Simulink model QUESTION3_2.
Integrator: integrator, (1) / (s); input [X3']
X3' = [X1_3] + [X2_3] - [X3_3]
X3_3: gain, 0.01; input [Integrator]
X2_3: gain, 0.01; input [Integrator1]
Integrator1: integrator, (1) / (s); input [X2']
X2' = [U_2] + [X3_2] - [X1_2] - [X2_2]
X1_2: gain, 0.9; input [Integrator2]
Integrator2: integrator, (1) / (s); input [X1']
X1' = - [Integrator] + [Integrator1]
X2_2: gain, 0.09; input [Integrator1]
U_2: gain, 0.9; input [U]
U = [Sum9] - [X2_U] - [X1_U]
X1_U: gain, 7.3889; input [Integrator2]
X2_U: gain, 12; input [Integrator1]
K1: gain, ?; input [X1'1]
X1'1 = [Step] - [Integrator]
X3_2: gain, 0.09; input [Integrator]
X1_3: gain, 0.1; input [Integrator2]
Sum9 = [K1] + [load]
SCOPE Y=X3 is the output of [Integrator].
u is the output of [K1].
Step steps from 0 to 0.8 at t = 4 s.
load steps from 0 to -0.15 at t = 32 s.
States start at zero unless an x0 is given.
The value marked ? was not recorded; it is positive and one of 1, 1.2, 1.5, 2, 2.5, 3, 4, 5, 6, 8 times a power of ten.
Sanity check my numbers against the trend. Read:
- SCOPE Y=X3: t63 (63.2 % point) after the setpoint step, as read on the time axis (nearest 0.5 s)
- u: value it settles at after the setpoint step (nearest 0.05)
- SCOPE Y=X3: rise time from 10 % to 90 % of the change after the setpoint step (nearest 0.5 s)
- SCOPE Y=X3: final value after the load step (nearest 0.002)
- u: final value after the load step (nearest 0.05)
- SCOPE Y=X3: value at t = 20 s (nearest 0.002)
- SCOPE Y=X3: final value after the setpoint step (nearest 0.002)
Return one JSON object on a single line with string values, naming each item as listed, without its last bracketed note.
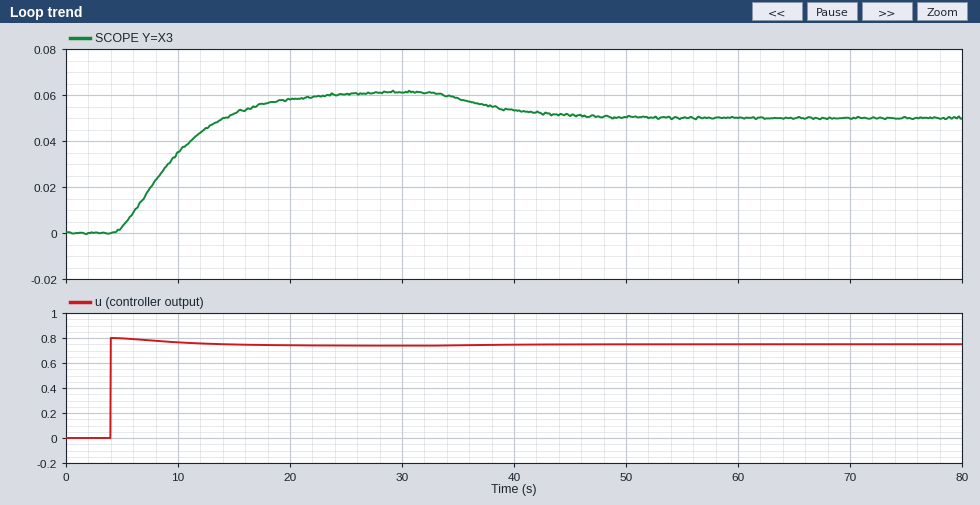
{"SCOPE Y=X3: t63 (63.2 % point) after the setpoint step, as read on the time axis": "11.0 s", "u: value it settles at after the setpoint step": "0.75", "SCOPE Y=X3: rise time from 10 % to 90 % of the change after the setpoint step": "11.5 s", "SCOPE Y=X3: final value after the load step": "0.050", "u: final value after the load step": "0.75", "SCOPE Y=X3: value at t = 20 s": "0.058", "SCOPE Y=X3: final value after the setpoint step": "0.062"}
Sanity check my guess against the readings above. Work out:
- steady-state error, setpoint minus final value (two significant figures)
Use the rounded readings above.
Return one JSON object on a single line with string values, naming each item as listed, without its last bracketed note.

{"steady-state error, setpoint minus final value": "0.74"}
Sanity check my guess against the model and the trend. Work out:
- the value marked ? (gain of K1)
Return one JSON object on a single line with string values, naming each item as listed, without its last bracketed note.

{"the value marked ?": "1"}
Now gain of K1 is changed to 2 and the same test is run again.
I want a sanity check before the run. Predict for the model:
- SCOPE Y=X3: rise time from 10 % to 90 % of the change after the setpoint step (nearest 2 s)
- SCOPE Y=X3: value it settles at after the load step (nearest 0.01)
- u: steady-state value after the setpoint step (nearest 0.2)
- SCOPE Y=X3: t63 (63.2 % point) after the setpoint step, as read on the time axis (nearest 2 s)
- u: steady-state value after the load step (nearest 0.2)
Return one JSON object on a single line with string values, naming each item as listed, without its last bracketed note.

{"SCOPE Y=X3: rise time from 10 % to 90 % of the change after the setpoint step": "10 s", "SCOPE Y=X3: value it settles at after the load step": "0.10", "u: steady-state value after the setpoint step": "1.4", "SCOPE Y=X3: t63 (63.2 % point) after the setpoint step, as read on the time axis": "10 s", "u: steady-state value after the load step": "1.4"}
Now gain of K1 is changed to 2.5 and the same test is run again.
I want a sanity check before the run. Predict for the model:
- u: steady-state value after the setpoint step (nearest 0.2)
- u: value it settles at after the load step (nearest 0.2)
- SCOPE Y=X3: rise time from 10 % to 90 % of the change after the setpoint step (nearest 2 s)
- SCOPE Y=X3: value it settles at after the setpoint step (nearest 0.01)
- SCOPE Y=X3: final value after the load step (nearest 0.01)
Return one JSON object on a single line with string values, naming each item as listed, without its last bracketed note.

{"u: steady-state value after the setpoint step": "1.6", "u: value it settles at after the load step": "1.6", "SCOPE Y=X3: rise time from 10 % to 90 % of the change after the setpoint step": "10 s", "SCOPE Y=X3: value it settles at after the setpoint step": "0.14", "SCOPE Y=X3: final value after the load step": "0.13"}
